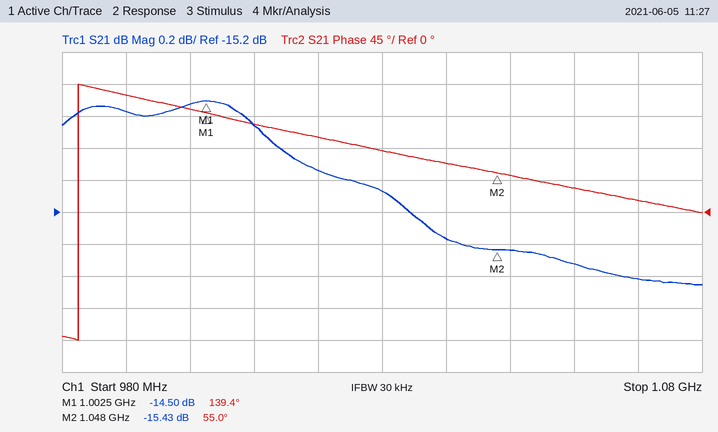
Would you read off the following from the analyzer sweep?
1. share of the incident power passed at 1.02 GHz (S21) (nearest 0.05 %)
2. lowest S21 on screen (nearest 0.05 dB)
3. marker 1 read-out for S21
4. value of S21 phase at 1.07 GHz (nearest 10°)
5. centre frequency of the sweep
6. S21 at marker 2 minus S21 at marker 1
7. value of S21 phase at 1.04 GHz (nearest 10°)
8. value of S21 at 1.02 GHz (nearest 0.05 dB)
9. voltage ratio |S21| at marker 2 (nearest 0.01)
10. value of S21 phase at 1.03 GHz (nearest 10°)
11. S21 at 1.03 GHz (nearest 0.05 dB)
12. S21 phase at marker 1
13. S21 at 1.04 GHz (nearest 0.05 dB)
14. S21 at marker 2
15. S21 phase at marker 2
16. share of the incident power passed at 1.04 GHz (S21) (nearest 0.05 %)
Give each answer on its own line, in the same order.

3.20 %
-15.65 dB
-14.50 dB
20°
1.03 GHz
-0.93 dB
70°
-14.95 dB
0.17
90°
-15.05 dB
139.4°
-15.35 dB
-15.43 dB
55.0°
2.90 %
